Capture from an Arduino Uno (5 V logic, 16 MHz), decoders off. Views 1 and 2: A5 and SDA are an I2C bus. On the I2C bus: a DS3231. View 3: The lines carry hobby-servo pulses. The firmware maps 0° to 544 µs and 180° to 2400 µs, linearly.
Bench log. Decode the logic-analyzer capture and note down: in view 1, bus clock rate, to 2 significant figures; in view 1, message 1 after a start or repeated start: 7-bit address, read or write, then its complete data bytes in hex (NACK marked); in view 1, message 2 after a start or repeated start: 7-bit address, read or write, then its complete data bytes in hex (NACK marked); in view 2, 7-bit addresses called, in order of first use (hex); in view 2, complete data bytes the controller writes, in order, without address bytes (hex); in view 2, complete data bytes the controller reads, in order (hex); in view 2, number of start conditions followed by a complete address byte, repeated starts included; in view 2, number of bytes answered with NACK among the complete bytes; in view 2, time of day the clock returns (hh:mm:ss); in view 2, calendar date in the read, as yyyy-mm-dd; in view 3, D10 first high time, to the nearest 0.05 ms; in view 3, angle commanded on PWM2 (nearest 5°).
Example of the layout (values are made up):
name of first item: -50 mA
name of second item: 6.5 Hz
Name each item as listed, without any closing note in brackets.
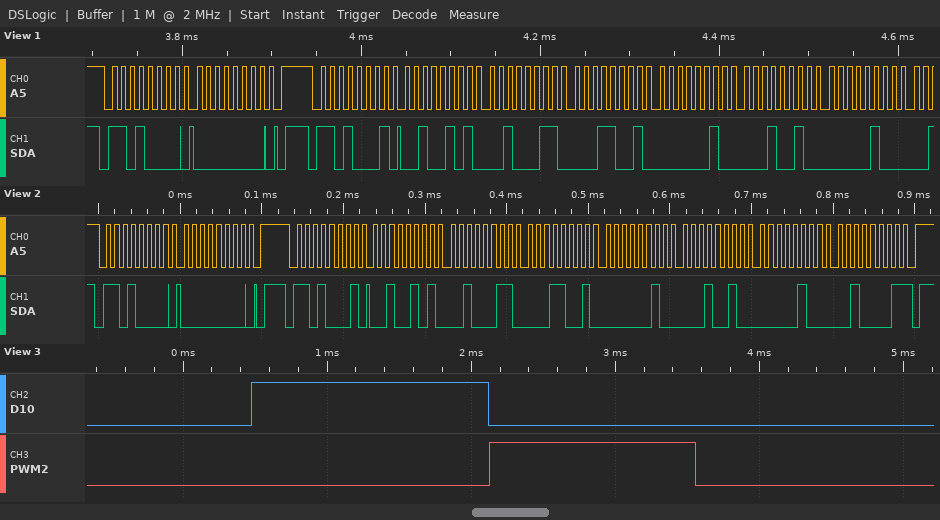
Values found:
in view 1, bus clock rate, to 2 significant figures: 100 kHz
in view 1, message 1 after a start or repeated start: 7-bit address, read or write, then its complete data bytes in hex: 0x68 write: 00
in view 1, message 2 after a start or repeated start: 7-bit address, read or write, then its complete data bytes in hex: 0x68 read: 25 23 19 02 12 04
in view 2, 7-bit addresses called, in order of first use: 0x68
in view 2, complete data bytes the controller writes, in order, without address bytes: 00
in view 2, complete data bytes the controller reads, in order: 25 23 19 02 12 04 21
in view 2, number of start conditions followed by a complete address byte, repeated starts included: 2
in view 2, number of bytes answered with NACK among the complete bytes: 1
in view 2, time of day the clock returns: 19:23:25
in view 2, calendar date in the read, as yyyy-mm-dd: 2021-04-12
in view 3, D10 first high time, to the nearest 0.05 ms: 1.65 ms
in view 3, angle commanded on PWM2: 85°
